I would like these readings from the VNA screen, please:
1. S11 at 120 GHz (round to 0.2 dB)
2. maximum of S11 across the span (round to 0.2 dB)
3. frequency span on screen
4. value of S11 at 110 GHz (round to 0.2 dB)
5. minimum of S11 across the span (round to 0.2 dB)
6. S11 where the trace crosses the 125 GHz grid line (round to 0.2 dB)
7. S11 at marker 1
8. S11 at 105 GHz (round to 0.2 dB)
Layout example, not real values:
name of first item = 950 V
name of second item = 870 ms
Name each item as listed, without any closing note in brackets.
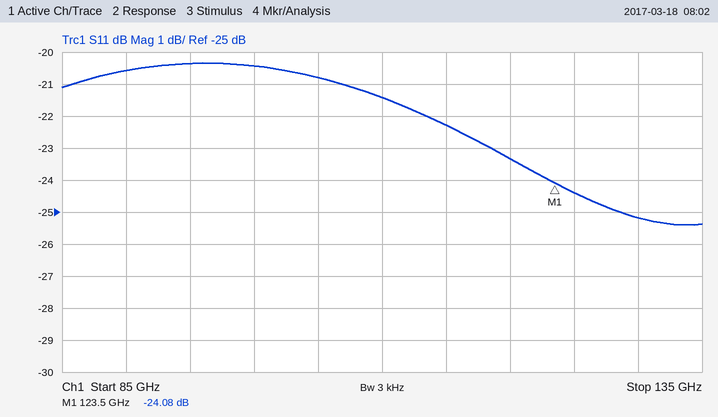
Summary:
S11 at 120 GHz = -23.4 dB
maximum of S11 across the span = -20.4 dB
frequency span on screen = 50 GHz
value of S11 at 110 GHz = -21.4 dB
minimum of S11 across the span = -25.4 dB
S11 where the trace crosses the 125 GHz grid line = -24.4 dB
S11 at marker 1 = -24.08 dB
S11 at 105 GHz = -20.8 dB
